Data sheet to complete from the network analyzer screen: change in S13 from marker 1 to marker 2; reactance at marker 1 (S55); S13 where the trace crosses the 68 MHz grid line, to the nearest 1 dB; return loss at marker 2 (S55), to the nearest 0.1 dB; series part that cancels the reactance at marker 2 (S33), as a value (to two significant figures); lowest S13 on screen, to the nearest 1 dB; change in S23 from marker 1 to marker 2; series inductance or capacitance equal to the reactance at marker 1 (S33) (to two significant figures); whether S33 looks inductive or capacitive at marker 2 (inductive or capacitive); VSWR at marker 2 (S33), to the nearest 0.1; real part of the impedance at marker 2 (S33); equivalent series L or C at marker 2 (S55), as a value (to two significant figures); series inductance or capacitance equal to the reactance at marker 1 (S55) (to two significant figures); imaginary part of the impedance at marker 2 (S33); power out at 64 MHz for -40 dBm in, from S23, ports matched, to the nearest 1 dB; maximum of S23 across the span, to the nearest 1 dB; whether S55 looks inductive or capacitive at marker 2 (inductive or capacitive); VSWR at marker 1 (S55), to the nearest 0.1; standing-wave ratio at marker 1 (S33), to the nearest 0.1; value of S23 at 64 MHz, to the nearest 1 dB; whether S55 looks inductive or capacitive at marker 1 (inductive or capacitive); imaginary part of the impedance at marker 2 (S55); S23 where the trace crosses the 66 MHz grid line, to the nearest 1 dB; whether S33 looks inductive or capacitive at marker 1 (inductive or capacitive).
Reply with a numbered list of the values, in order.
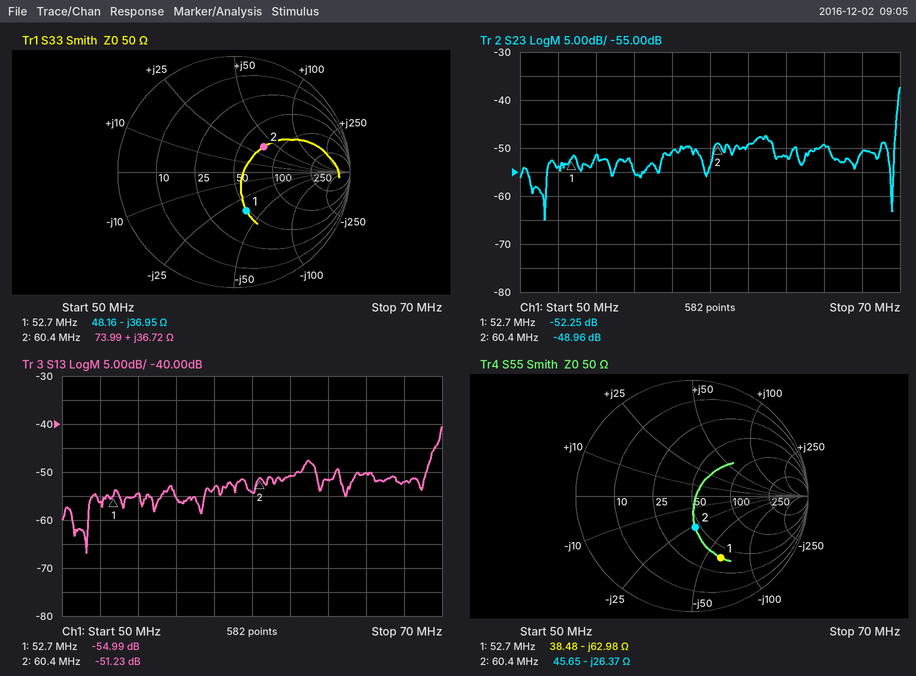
1. 3.76 dB
2. -62.98 Ω
3. -52 dB
4. 11.4 dB
5. 72 pF
6. -67 dB
7. 3.29 dB
8. 82 pF
9. inductive
10. 2.0
11. 73.99 Ω
12. 100 pF
13. 48 pF
14. +36.72 Ω
15. -92 dBm
16. -37 dB
17. capacitive
18. 3.9
19. 2.1
20. -52 dB
21. capacitive
22. -26.37 Ω
23. -49 dB
24. capacitive
